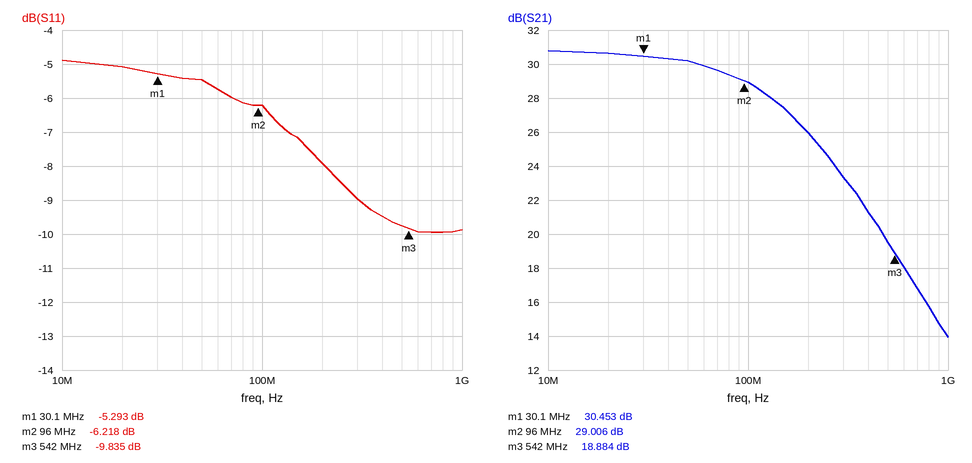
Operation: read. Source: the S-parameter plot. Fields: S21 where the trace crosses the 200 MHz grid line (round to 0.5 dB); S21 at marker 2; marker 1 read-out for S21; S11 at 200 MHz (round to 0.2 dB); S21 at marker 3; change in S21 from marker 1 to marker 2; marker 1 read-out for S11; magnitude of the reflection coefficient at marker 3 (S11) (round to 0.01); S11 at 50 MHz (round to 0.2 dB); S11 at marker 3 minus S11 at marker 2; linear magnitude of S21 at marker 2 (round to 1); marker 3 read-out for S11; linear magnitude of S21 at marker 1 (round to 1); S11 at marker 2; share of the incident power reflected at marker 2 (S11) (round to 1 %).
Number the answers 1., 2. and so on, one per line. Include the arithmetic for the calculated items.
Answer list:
1. 26.0 dB
2. 29.006 dB
3. 30.453 dB
4. -8.0 dB
5. 18.884 dB
6. 29.006 − (30.453) = -1.447 dB
7. -5.293 dB
8. 10^(-9.835/20) ≈ 0.32
9. -5.4 dB
10. -9.835 − (-6.218) = -3.617 dB
11. 10^(29.006/20) ≈ 28
12. -9.835 dB
13. 10^(30.453/20) ≈ 33
14. -6.218 dB
15. 10^(-6.218/10) ≈ 24 %
